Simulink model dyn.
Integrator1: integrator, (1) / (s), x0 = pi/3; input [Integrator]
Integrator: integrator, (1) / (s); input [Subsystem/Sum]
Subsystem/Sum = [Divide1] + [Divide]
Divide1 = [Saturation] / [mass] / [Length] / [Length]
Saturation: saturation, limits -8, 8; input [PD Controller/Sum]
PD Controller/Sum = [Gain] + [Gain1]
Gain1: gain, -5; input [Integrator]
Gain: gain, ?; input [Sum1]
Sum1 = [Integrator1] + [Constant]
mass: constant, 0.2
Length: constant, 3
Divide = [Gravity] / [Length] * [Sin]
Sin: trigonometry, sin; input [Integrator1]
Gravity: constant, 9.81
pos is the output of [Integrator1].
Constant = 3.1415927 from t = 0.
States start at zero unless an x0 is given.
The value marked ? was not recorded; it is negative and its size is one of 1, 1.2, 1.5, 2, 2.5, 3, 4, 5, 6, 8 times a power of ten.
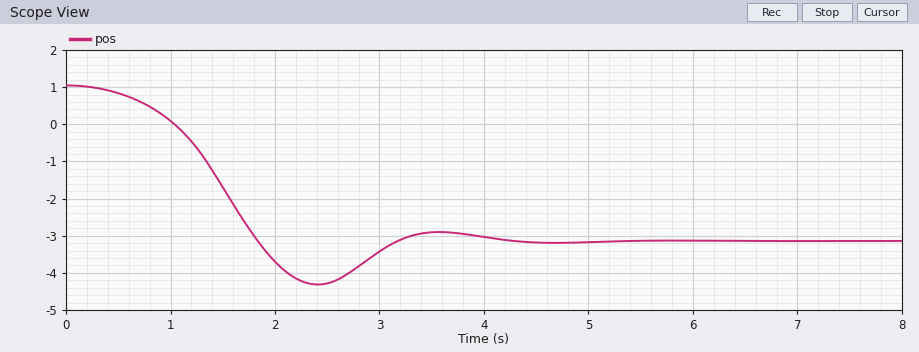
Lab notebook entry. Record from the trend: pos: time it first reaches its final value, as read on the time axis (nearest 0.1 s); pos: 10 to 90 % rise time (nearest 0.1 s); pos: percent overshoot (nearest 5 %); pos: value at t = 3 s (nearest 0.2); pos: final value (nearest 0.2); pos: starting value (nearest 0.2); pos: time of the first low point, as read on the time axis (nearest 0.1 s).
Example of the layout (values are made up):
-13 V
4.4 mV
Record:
1.8 s
1.0 s
30 %
-3.4
-3.2
1.0
2.4 s
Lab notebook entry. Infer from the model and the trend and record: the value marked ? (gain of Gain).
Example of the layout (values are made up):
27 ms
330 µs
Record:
-12
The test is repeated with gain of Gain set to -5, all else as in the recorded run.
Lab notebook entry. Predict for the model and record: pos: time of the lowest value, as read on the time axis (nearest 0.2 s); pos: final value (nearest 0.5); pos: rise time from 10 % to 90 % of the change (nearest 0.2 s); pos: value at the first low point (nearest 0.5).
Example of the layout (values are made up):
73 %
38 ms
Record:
2.8 s
-3.0
1.4 s
-3.5
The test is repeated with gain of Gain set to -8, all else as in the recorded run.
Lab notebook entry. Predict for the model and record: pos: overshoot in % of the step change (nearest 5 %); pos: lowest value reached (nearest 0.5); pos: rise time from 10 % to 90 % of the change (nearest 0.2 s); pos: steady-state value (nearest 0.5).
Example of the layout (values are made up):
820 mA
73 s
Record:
15 %
-4.0
1.2 s
-3.0
